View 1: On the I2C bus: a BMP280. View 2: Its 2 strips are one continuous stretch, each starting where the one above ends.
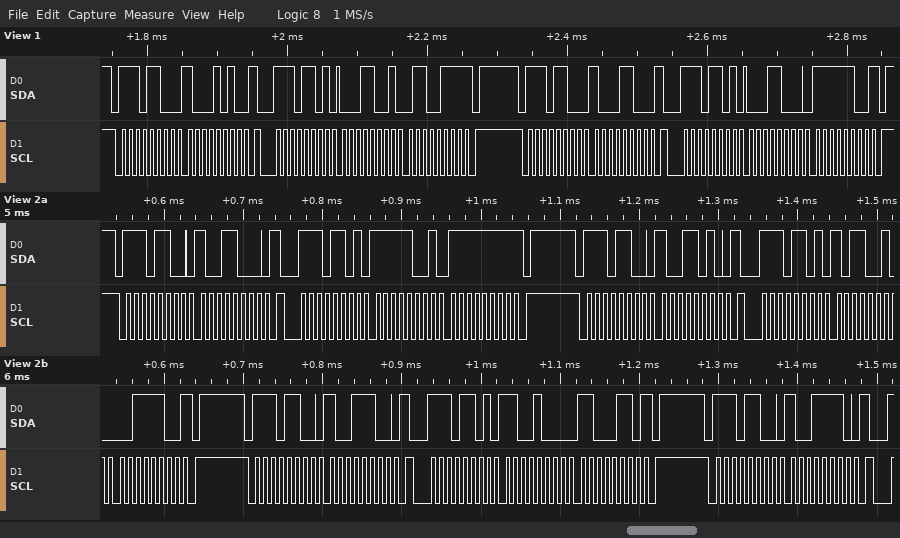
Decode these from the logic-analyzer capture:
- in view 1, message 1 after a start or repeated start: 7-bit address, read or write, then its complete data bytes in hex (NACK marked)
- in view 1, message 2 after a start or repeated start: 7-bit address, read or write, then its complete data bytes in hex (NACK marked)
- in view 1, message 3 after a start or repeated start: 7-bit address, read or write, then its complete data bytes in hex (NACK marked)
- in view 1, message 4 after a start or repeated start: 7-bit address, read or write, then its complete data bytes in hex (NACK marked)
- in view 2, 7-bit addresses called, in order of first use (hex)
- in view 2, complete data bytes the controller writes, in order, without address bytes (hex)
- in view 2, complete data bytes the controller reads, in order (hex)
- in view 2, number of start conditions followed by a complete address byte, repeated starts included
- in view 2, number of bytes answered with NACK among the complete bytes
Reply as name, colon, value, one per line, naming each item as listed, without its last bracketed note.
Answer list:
in view 1, message 1 after a start or repeated start: 7-bit address, read or write, then its complete data bytes in hex: 0x76 write: 8A
in view 1, message 2 after a start or repeated start: 7-bit address, read or write, then its complete data bytes in hex: 0x76 read: 19 67 NACK
in view 1, message 3 after a start or repeated start: 7-bit address, read or write, then its complete data bytes in hex: 0x76 write: 8C
in view 1, message 4 after a start or repeated start: 7-bit address, read or write, then its complete data bytes in hex: 0x76 read: 18 FC NACK
in view 2, 7-bit addresses called, in order of first use: 0x76
in view 2, complete data bytes the controller writes, in order, without address bytes: 98 9A 9C 9E
in view 2, complete data bytes the controller reads, in order: F9 FF B2 3C C8 C6
in view 2, number of start conditions followed by a complete address byte, repeated starts included: 7
in view 2, number of bytes answered with NACK among the complete bytes: 3
